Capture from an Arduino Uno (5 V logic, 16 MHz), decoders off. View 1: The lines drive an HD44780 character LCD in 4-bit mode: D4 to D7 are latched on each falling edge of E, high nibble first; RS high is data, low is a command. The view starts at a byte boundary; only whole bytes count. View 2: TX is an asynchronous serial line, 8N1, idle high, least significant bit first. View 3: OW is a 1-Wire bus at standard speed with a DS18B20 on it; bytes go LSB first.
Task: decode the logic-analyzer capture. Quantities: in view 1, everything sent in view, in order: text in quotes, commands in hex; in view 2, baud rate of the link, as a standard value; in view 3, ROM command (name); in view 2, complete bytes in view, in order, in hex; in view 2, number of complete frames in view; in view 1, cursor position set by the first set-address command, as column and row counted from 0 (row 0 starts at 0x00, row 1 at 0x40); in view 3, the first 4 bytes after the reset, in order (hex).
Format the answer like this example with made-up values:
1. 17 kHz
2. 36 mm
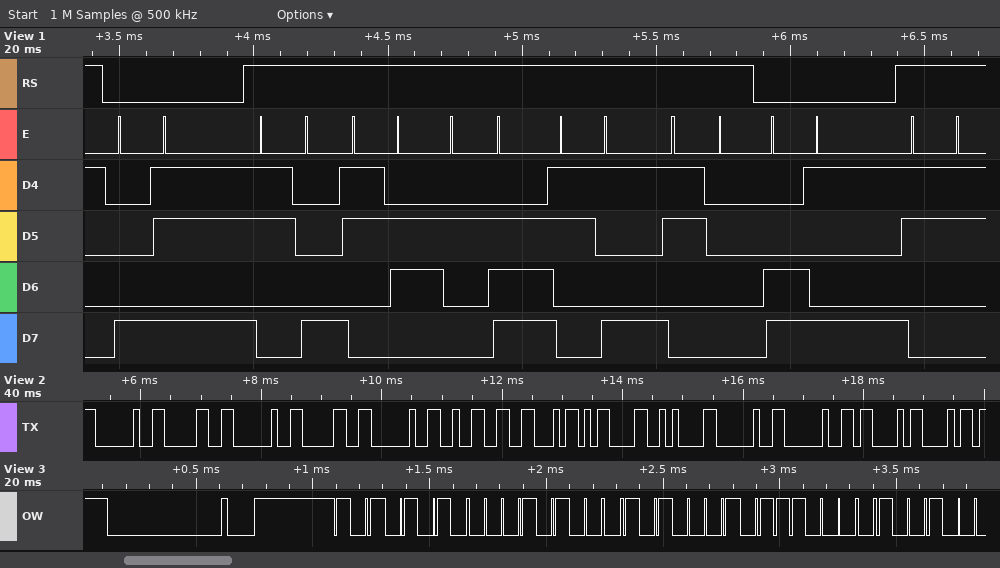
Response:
1. 0x8B "86.90" 0xC9 "3"
2. 9600 baud
3. Match ROM
4. 20 30 20 30 20 32 46 0D 0A 20 20 43 68
5. 13
6. column 11, row 0
7. 55 28 8A 0E
